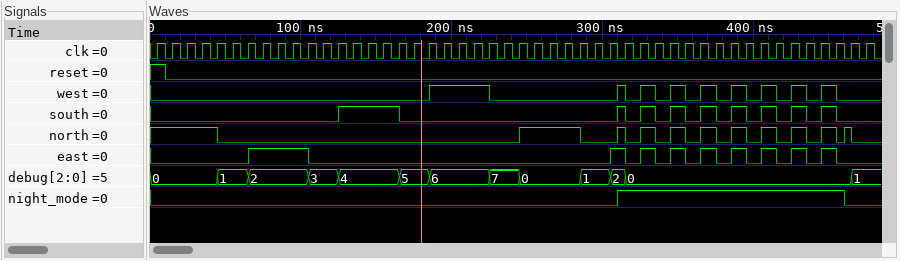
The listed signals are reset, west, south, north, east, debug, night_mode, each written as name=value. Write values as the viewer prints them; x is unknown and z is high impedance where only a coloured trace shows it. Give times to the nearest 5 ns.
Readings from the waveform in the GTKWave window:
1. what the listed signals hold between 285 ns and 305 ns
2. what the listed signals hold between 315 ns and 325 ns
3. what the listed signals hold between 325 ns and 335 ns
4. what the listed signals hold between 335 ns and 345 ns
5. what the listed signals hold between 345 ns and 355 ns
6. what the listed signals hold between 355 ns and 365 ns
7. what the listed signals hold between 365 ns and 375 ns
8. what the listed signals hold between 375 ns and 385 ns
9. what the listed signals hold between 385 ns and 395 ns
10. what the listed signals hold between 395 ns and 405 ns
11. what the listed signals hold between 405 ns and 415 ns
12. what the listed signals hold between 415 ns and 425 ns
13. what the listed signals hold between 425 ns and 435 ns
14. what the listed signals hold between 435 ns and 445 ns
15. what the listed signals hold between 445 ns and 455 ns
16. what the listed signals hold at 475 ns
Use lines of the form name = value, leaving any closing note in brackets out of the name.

what the listed signals hold between 285 ns and 305 ns = reset=0, west=0, south=0, north=0, east=0, debug=1, night_mode=0
what the listed signals hold between 315 ns and 325 ns = reset=0, west=0, south=0, north=0, east=0, debug=0, night_mode=1
what the listed signals hold between 325 ns and 335 ns = reset=0, west=1, south=1, north=1, east=1, debug=0, night_mode=1
what the listed signals hold between 335 ns and 345 ns = reset=0, west=0, south=0, north=0, east=0, debug=0, night_mode=1
what the listed signals hold between 345 ns and 355 ns = reset=0, west=1, south=1, north=1, east=1, debug=0, night_mode=1
what the listed signals hold between 355 ns and 365 ns = reset=0, west=0, south=0, north=0, east=0, debug=0, night_mode=1
what the listed signals hold between 365 ns and 375 ns = reset=0, west=1, south=1, north=1, east=1, debug=0, night_mode=1
what the listed signals hold between 375 ns and 385 ns = reset=0, west=0, south=0, north=0, east=0, debug=0, night_mode=1
what the listed signals hold between 385 ns and 395 ns = reset=0, west=1, south=1, north=1, east=1, debug=0, night_mode=1
what the listed signals hold between 395 ns and 405 ns = reset=0, west=0, south=0, north=0, east=0, debug=0, night_mode=1
what the listed signals hold between 405 ns and 415 ns = reset=0, west=1, south=1, north=1, east=1, debug=0, night_mode=1
what the listed signals hold between 415 ns and 425 ns = reset=0, west=0, south=0, north=0, east=0, debug=0, night_mode=1
what the listed signals hold between 425 ns and 435 ns = reset=0, west=1, south=1, north=1, east=1, debug=0, night_mode=1
what the listed signals hold between 435 ns and 445 ns = reset=0, west=0, south=0, north=0, east=0, debug=0, night_mode=1
what the listed signals hold between 445 ns and 455 ns = reset=0, west=1, south=1, north=1, east=1, debug=0, night_mode=1
what the listed signals hold at 475 ns = reset=0, west=0, south=0, north=0, east=0, debug=1, night_mode=0
